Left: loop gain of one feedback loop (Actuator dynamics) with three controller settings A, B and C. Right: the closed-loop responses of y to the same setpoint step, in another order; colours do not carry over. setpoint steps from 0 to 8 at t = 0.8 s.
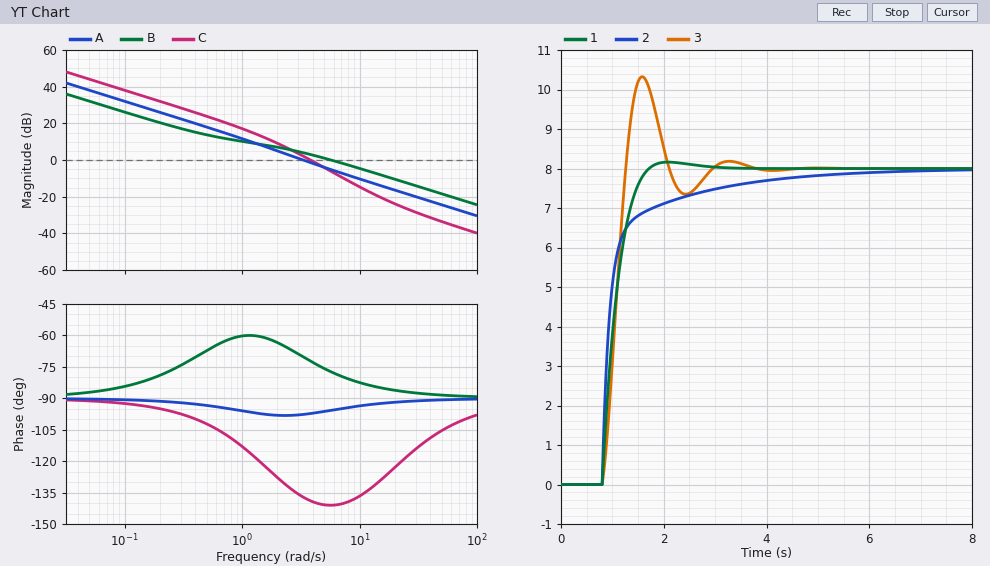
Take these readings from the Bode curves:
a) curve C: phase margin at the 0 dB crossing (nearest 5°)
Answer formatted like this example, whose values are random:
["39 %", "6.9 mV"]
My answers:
["40°"]
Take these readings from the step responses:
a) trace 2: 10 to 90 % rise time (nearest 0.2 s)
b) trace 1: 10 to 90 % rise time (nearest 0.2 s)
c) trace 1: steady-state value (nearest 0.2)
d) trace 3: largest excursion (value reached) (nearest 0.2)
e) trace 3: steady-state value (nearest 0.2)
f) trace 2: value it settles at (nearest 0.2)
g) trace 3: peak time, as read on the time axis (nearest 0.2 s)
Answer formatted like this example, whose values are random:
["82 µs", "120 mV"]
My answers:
["1.4 s", "0.6 s", "8.0", "10.4", "8.0", "8.0", "1.6 s"]
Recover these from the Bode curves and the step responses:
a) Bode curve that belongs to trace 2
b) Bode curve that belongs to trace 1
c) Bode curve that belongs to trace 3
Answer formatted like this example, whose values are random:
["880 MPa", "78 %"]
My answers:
["B", "A", "C"]
